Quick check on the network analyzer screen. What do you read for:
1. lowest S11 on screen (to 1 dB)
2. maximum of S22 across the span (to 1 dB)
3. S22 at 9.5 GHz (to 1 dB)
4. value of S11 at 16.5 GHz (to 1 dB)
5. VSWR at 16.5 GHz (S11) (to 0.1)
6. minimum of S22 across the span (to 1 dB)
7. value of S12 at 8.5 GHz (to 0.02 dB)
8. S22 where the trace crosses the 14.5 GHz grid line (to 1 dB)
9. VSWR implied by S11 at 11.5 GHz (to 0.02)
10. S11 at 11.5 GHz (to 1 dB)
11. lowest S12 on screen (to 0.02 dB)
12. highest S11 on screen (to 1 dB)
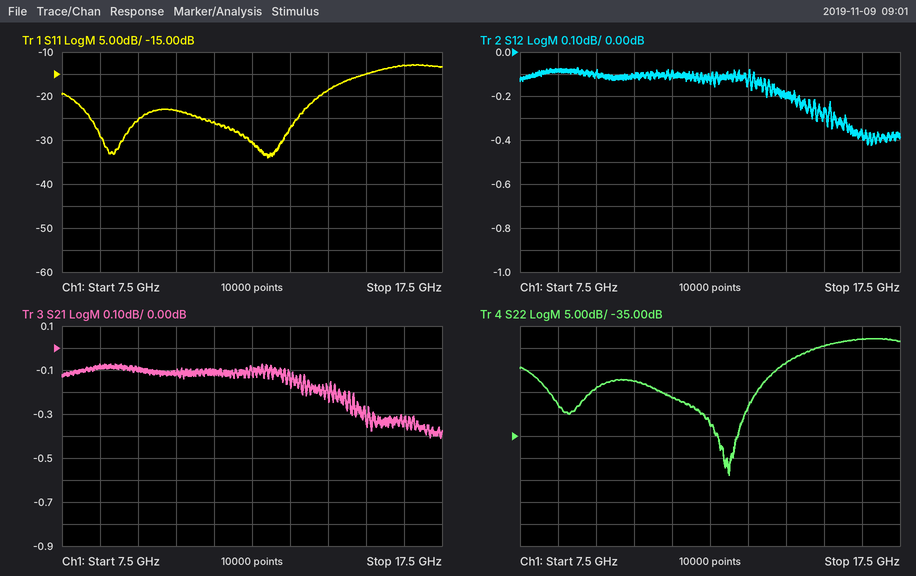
-34 dB
-13 dB
-24 dB
-13 dB
1.6
-44 dB
-0.08 dB
-18 dB
1.10
-26 dB
-0.42 dB
-13 dB
